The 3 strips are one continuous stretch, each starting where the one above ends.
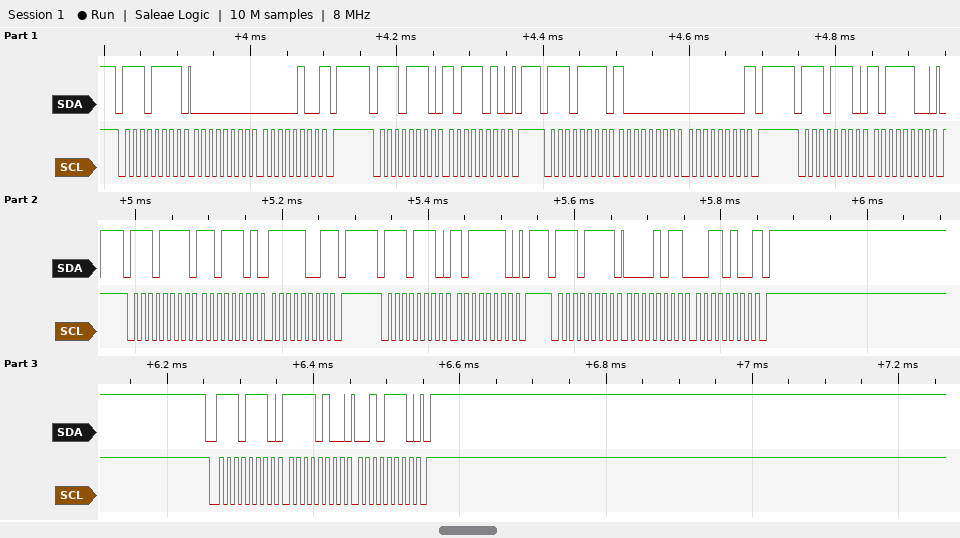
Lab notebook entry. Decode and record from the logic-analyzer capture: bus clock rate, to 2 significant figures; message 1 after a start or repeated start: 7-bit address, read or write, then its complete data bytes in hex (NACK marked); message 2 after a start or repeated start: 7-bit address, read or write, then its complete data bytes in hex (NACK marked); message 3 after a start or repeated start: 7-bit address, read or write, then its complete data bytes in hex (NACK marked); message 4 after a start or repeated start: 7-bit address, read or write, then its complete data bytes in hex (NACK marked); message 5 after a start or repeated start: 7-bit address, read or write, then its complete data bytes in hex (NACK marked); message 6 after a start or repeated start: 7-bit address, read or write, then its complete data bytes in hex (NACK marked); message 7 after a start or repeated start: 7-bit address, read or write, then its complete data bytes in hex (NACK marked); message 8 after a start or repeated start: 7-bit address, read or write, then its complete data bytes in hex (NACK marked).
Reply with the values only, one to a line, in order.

100 kHz
0x77 read: 00 04 NACK
0x77 write: BA
0x77 read: 80 00 NACK
0x77 write: BC
0x77 read: DD F9 NACK
0x77 write: BE
0x77 read: 0B 34 NACK
0x77 write: F4 2E
